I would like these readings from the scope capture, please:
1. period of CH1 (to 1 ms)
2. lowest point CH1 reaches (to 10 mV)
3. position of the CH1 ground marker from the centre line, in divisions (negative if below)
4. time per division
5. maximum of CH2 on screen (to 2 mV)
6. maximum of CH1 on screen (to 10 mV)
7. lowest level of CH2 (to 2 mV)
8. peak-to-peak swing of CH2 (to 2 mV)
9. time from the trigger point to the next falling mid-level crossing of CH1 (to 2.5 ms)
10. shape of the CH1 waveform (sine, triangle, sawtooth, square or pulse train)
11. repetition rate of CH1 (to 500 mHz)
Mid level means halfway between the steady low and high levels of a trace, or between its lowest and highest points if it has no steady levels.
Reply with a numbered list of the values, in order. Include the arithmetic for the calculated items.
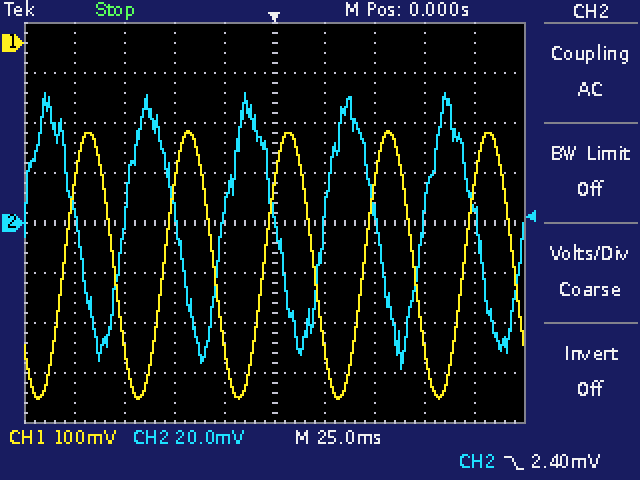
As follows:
1. 50 ms
2. -710 mV
3. +3.6 div
4. 25 ms
5. 52 mV
6. -180 mV
7. -58 mV
8. 52 mV − (-58 mV) = 110 mV
9. 20.0 ms
10. sine
11. 1 / 50 ms ≈ 20.0 Hz
